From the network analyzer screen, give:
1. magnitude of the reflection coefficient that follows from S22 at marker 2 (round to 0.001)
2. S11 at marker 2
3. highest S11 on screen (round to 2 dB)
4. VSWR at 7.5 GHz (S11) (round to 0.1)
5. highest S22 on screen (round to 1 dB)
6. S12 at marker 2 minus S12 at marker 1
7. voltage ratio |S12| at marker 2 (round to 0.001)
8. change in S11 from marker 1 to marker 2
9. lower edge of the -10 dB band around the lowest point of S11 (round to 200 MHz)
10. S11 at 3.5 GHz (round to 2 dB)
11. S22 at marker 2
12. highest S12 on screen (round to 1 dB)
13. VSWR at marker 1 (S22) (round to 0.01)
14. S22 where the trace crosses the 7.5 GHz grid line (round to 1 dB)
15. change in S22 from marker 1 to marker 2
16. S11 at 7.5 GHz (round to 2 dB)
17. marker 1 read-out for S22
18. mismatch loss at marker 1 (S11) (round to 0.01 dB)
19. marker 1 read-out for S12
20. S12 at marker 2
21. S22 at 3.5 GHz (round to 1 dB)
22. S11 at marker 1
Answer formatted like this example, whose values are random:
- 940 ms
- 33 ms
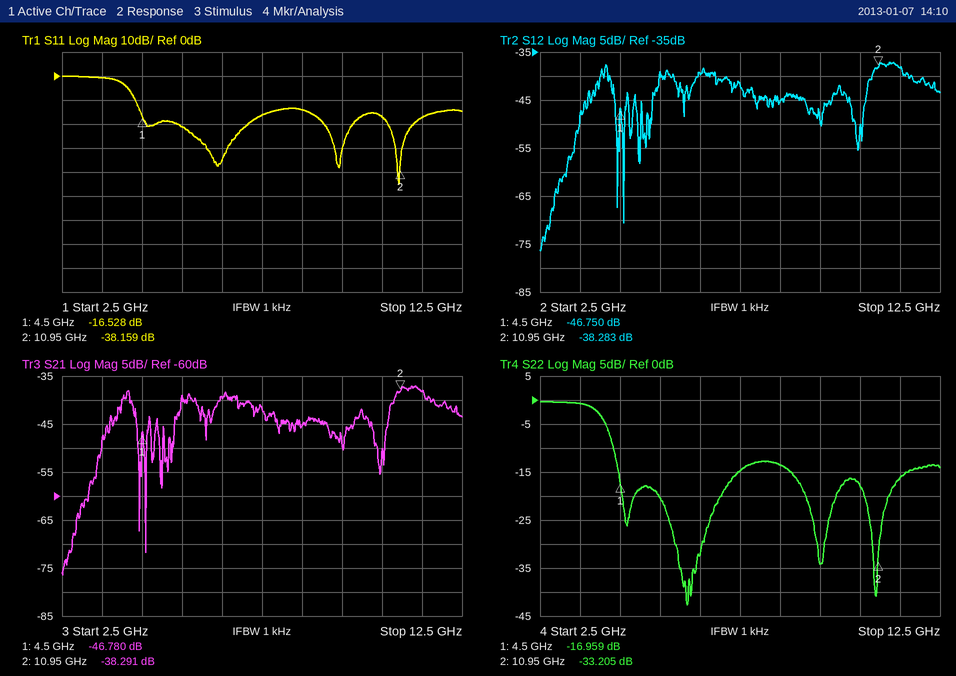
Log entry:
- 0.022
- -38.159 dB
- 0 dB
- 1.4
- 0 dB
- 8.467 dB
- 0.012
- -21.631 dB
- 4.4 GHz
- 0 dB
- -33.205 dB
- -37 dB
- 1.33
- -15 dB
- -16.246 dB
- -16 dB
- -16.959 dB
- 0.10 dB
- -46.750 dB
- -38.283 dB
- -1 dB
- -16.528 dB
